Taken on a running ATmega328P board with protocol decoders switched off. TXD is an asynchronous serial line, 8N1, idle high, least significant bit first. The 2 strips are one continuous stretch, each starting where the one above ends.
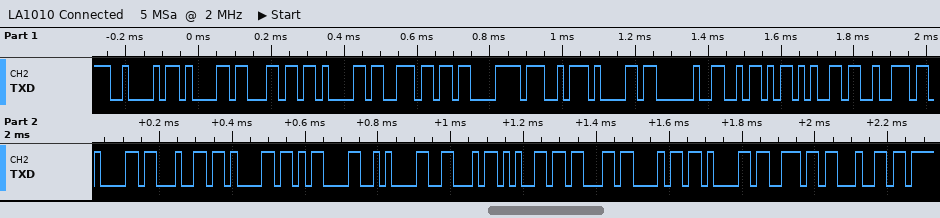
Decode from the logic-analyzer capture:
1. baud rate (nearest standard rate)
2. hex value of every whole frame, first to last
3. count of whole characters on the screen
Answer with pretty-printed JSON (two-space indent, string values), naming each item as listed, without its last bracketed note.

{
  "baud rate": "57600 baud",
  "hex value of every whole frame, first to last": "0x42 0x61 0x6C 0x61 0x6E 0xC3 0xA7 0x61 0x20 0x5A 0x65 0x72 0x61 0x64 0x61 0x0D 0x0A 0x46 0x65 0x63 0x68 0x61 0x6E 0x64",
  "count of whole characters on the screen": "24"
}
